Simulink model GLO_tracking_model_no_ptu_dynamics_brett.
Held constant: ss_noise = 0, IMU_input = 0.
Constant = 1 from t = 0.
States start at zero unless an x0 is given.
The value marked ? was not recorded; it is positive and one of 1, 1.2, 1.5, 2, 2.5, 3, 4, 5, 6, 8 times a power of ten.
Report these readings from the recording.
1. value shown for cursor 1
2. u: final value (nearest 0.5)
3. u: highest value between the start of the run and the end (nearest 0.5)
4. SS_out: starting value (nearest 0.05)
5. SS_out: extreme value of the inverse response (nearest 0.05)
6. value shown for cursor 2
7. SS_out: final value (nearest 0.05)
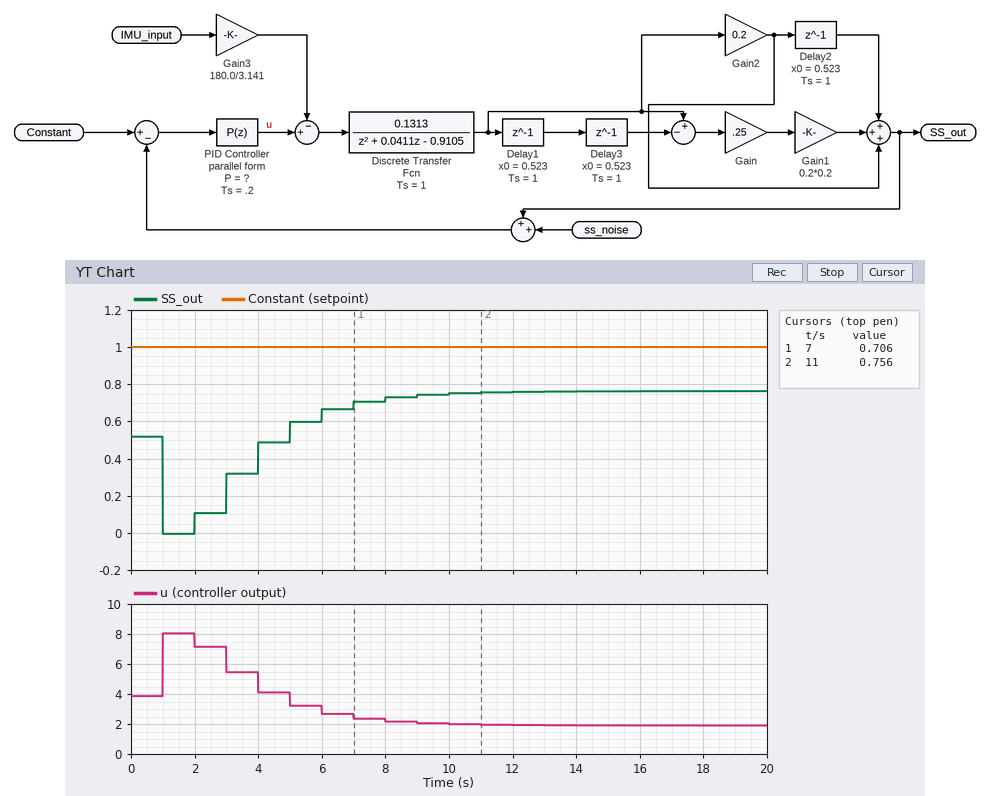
0.706
2.0
8.0
0.50
0.00
0.756
0.75
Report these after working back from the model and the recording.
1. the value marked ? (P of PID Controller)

8
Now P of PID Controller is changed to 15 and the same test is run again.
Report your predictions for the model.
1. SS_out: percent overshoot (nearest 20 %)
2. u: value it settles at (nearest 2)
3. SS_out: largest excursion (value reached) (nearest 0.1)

40 %
2
1.0
